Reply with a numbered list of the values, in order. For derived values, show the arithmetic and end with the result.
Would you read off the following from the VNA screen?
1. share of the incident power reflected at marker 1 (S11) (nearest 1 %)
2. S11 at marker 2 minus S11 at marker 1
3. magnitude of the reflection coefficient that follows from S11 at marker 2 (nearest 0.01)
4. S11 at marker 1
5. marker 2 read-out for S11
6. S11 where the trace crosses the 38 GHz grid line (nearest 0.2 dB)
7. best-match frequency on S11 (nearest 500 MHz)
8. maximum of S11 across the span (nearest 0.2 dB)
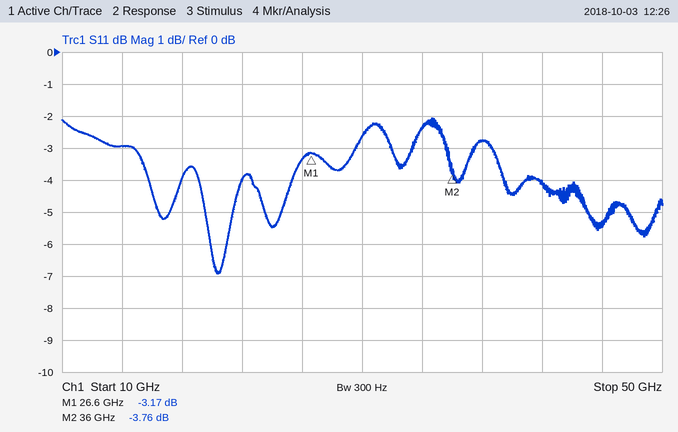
1. 10^(-3.17/10) ≈ 48 %
2. -3.76 − (-3.17) = -0.59 dB
3. 10^(-3.76/20) ≈ 0.65
4. -3.17 dB
5. -3.76 dB
6. -2.8 dB
7. 20.5 GHz
8. -2.0 dB
